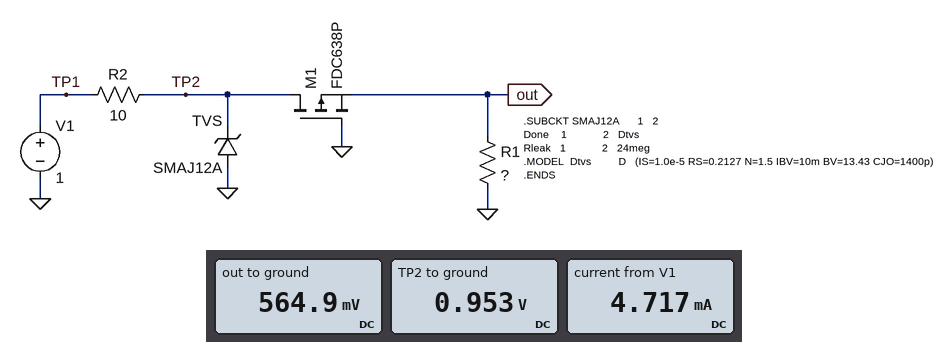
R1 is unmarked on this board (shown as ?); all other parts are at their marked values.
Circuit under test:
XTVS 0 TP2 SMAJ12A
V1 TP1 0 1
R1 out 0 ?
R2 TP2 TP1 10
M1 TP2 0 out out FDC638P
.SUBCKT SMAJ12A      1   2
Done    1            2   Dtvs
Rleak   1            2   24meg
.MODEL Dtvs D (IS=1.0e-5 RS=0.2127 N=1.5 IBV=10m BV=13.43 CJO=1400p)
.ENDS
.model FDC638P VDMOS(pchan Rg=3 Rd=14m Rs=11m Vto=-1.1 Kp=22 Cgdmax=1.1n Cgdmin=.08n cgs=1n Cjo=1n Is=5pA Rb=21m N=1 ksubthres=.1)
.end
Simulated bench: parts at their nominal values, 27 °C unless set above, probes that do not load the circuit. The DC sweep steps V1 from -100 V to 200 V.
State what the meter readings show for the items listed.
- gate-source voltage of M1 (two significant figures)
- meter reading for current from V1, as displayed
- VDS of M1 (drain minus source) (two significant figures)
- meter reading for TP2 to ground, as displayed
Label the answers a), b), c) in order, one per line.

a) -560 mV
b) 4.717 mA
c) 390 mV
d) 0.953 V
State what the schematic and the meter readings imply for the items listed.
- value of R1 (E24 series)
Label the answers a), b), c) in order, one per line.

a) 120 Ω
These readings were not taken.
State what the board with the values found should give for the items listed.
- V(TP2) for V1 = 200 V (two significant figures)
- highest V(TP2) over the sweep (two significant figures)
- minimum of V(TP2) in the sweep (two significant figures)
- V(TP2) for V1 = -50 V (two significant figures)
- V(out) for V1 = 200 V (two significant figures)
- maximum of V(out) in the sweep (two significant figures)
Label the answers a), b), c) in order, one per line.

a) 18 V
b) 18 V
c) -2.6 V
d) -1.5 V
e) 18 V
f) 18 V
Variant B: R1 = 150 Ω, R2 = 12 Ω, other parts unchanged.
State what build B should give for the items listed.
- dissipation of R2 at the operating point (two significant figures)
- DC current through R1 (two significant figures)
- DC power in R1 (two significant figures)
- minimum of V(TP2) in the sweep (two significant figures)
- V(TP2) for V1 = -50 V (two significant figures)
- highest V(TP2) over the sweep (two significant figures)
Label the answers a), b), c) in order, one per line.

a) 220 µW
b) 4.3 mA
c) 2.8 mW
d) -2.3 V
e) -1.4 V
f) 17 V
